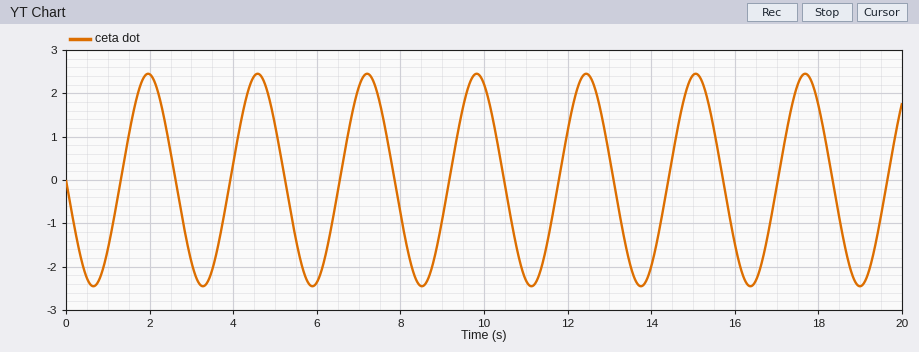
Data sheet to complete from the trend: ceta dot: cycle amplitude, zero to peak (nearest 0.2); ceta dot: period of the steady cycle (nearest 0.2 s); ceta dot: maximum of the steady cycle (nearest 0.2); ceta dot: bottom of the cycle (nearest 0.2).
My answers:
2.4
2.6 s
2.4
-2.4
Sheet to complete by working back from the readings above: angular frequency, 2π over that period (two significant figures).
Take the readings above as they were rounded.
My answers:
2.4 rad/s
